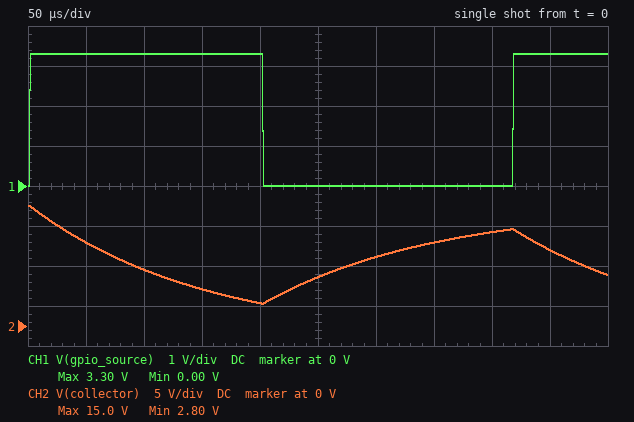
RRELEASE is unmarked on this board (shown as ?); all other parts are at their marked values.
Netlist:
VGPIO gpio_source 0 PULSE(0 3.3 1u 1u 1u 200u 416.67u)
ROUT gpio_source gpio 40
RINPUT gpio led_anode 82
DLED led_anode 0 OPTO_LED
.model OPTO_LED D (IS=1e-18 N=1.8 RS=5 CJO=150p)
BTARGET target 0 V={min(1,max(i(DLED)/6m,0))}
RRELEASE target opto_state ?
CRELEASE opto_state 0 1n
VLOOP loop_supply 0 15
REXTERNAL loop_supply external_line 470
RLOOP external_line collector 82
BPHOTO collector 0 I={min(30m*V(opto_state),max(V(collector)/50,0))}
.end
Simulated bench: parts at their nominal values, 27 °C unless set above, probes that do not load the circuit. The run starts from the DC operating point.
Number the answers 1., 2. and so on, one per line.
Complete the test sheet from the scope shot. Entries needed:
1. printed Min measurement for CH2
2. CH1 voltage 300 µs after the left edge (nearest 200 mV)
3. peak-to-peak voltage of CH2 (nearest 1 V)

1. 2.80 V
2. 0 V
3. 12 V
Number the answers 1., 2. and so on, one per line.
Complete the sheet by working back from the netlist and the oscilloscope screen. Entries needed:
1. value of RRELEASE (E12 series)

1. 150 kΩ
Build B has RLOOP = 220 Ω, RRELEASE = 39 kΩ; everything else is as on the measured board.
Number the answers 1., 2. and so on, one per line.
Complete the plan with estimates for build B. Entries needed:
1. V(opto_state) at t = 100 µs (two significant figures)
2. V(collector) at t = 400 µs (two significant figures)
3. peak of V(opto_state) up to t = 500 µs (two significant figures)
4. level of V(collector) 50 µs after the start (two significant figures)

1. 920 mV
2. 15 V
3. 990 mV
4. 1.0 V
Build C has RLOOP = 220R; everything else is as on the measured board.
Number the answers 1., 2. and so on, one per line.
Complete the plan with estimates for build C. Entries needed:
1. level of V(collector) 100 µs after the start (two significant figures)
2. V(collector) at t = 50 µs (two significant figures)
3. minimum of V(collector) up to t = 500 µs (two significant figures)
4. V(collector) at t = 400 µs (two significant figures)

1. 5.0 V
2. 9.3 V
3. 1.0 V
4. 11 V
